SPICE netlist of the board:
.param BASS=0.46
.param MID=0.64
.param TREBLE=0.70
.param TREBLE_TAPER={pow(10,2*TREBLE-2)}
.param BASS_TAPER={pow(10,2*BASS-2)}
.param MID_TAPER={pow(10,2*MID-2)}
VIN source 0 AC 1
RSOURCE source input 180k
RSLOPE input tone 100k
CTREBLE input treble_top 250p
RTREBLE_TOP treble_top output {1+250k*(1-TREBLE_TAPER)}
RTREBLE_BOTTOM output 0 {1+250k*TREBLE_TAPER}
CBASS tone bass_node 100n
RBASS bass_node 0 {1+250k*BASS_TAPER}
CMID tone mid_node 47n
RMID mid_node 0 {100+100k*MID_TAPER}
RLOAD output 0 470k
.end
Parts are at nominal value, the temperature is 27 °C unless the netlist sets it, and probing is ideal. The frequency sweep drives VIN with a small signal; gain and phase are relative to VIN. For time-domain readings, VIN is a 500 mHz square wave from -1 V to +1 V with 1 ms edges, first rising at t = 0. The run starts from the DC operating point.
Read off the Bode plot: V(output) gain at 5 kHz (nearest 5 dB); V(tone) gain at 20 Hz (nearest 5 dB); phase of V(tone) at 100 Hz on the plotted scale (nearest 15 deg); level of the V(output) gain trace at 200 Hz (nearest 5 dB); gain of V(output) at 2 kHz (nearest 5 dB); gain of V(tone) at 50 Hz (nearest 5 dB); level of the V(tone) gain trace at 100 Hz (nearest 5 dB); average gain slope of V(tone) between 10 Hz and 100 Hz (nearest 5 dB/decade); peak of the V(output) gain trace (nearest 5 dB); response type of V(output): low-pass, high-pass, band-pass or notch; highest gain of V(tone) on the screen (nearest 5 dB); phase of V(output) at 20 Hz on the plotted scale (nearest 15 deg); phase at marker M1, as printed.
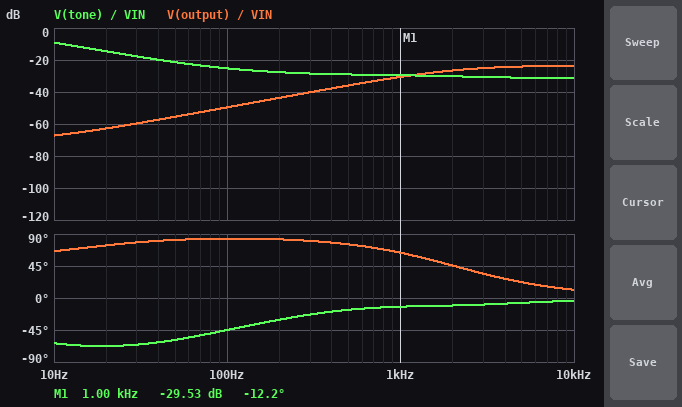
-25 dB
-15 dB
-45 deg
-45 dB
-25 dB
-20 dB
-25 dB
-15 dB/decade
-25 dB
high-pass
-10 dB
75 deg
-12.2 deg
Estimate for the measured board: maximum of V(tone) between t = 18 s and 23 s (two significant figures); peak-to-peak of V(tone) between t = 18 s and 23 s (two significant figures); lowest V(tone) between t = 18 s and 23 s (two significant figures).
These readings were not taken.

1.0 V
2.0 V
-1.0 V
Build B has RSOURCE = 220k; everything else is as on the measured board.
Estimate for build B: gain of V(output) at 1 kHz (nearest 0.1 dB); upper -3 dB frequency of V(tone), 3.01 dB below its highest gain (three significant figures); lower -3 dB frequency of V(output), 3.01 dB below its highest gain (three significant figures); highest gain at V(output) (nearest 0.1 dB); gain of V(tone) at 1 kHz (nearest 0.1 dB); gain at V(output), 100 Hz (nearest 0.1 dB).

-31.7 dB
3.27 Hz
2.02 kHz
-24.7 dB
-30.7 dB
-50.7 dB
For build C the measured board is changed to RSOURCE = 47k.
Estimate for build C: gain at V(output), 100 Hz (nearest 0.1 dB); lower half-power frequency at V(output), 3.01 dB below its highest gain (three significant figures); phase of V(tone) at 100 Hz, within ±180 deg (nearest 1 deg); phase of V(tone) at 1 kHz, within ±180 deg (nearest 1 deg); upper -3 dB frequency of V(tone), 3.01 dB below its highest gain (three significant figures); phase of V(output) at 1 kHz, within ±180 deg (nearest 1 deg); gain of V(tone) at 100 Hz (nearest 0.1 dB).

-44.3 dB
2.31 kHz
-43 deg
-9 deg
6.87 Hz
66 deg
-19.9 dB
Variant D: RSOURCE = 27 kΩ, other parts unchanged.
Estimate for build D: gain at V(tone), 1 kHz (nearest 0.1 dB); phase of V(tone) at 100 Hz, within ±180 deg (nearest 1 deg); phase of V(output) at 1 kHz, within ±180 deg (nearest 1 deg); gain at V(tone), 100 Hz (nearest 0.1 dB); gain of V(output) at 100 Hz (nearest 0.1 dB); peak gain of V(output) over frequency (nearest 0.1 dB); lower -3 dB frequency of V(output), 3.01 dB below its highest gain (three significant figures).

-22.8 dB
-42 deg
67 deg
-18.8 dB
-43.1 dB
-15.5 dB
2.41 kHz
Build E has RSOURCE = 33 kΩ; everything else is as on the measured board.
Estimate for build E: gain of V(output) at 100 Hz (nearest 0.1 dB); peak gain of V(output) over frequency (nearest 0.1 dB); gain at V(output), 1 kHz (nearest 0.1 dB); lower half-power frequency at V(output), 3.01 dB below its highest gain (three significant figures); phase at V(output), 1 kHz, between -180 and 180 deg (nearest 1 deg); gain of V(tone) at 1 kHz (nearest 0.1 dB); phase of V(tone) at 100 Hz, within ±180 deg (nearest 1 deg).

-43.5 dB
-16.0 dB
-24.2 dB
2.38 kHz
67 deg
-23.2 dB
-42 deg
